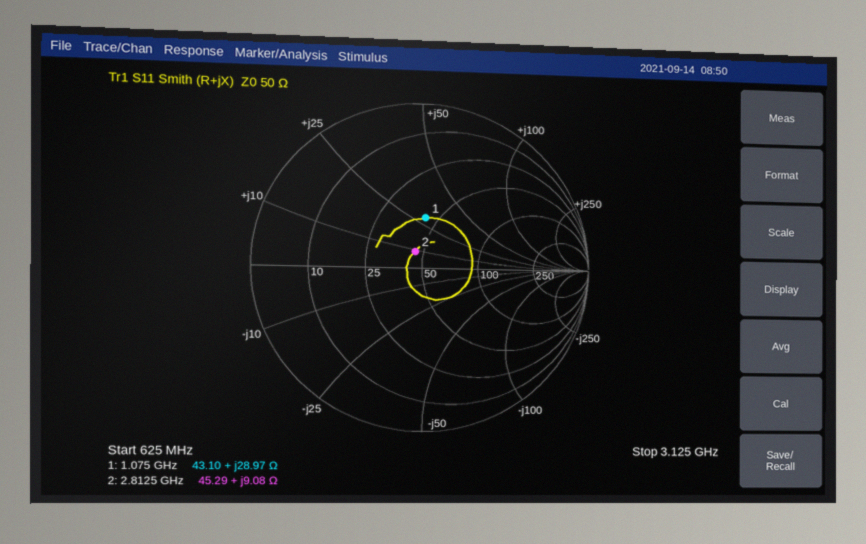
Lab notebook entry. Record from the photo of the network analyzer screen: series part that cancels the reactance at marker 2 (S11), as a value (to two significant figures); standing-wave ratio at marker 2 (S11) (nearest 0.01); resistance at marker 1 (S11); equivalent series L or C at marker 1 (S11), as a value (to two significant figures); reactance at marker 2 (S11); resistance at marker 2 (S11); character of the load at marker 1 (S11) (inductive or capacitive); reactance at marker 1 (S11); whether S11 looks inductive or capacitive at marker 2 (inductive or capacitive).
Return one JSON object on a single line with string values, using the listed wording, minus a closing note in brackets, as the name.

{"series part that cancels the reactance at marker 2 (S11), as a value": "6.2 pF", "standing-wave ratio at marker 2 (S11)": "1.24", "resistance at marker 1": "43.10 Ω", "equivalent series L or C at marker 1 (S11), as a value": "4.3 nH", "reactance at marker 2": "+9.08 Ω", "resistance at marker 2": "45.29 Ω", "character of the load at marker 1 (S11)": "inductive", "reactance at marker 1": "+28.97 Ω", "whether S11 looks inductive or capacitive at marker 2": "inductive"}
